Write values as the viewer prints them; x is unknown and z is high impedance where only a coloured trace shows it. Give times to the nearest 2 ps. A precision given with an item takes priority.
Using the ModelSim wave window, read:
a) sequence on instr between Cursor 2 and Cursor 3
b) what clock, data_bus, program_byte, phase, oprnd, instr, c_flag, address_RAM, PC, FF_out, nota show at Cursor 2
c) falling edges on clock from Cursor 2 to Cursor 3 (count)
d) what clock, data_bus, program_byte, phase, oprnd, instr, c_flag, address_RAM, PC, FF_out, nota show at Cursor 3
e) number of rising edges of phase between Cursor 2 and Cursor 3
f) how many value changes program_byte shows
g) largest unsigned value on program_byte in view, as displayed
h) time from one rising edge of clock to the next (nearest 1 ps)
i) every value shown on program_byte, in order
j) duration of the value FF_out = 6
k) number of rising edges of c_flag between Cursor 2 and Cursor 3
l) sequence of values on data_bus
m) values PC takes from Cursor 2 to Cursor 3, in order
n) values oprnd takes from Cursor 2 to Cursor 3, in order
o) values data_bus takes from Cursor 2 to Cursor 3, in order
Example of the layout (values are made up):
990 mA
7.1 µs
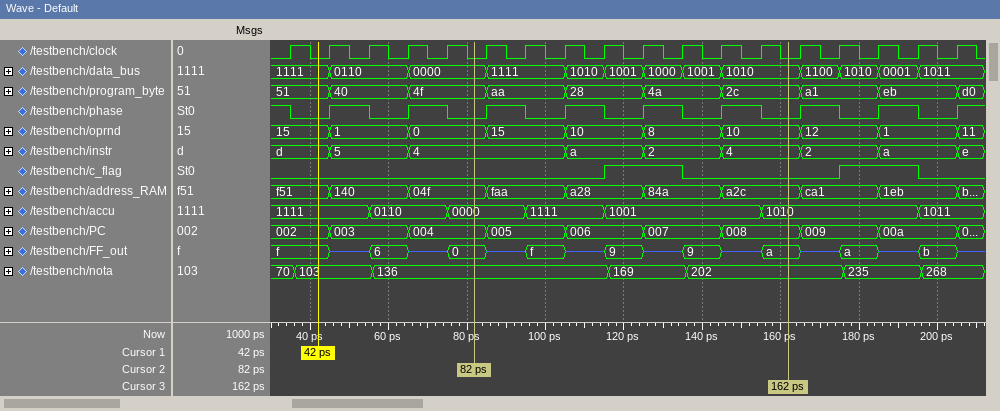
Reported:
4, a, 2, 4
clock=0, data_bus=0000, program_byte=4f, phase=0, oprnd=0, instr=4, c_flag=0, address_RAM=04f, PC=004, FF_out=0, nota=136
8
clock=0, data_bus=1010, program_byte=2c, phase=0, oprnd=10, instr=4, c_flag=0, address_RAM=a2c, PC=008, FF_out=a, nota=202
4
9
eb
10 ps
51, 40, 4f, aa, 28, 4a, 2c, a1, eb, d0
10 ps
1
1111, 0110, 0000, 1111, 1010, 1001, 1000, 1001, 1010, 1100, 1010, 0001, 1011
004, 005, 006, 007, 008
0, 15, 10, 8, 10
0000, 1111, 1010, 1001, 1000, 1001, 1010
